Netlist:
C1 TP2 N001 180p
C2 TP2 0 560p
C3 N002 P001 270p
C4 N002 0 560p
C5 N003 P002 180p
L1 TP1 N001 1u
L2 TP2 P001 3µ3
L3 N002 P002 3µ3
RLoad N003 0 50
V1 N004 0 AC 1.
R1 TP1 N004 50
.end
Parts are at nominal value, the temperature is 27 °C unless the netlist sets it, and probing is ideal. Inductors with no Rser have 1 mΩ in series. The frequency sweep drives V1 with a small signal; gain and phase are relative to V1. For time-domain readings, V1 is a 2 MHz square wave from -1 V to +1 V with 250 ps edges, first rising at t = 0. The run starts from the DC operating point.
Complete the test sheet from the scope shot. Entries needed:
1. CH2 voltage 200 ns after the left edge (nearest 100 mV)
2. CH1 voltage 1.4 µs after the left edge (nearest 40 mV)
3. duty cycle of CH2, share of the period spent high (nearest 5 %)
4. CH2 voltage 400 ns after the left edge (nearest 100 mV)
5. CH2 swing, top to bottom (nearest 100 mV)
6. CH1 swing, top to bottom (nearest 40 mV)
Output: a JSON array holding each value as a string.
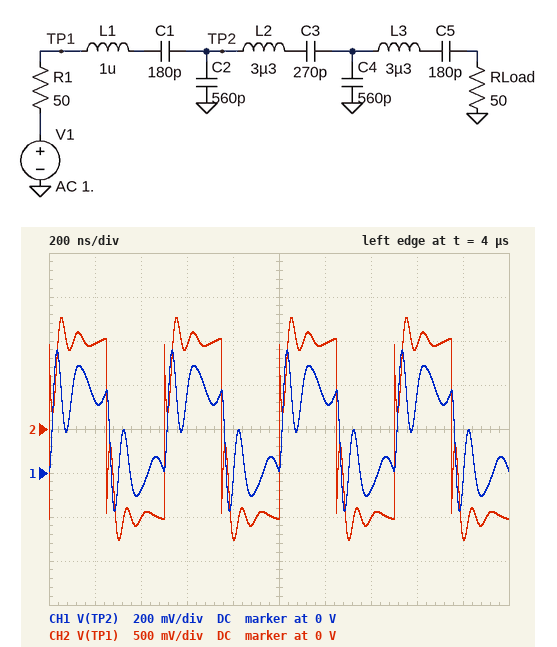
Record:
["1.0 V", "-80 mV", "50 %", "-1.0 V", "2.5 V", "720 mV"]
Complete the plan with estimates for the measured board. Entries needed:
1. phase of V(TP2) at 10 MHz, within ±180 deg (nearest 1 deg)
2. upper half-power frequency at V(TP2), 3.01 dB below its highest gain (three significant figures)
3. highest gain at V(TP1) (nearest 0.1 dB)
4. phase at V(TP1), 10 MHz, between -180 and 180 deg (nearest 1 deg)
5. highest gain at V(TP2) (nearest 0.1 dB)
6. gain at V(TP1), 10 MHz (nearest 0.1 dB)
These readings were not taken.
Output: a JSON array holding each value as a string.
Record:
["-38 deg", "15.6 MHz", "0 dB", "-38 deg", "-5.9 dB", "-2.1 dB"]
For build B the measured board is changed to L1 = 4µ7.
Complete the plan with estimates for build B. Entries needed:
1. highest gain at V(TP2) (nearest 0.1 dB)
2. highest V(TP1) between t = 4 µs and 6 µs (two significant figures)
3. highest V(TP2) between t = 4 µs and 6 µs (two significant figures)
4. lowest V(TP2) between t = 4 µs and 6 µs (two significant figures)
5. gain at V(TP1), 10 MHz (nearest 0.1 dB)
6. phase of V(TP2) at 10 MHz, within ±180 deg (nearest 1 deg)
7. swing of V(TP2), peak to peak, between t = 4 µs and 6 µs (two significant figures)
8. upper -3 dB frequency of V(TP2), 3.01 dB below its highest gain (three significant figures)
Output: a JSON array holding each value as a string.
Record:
["-3.0 dB", "1.3 V", "510 mV", "-130 mV", "-0.4 dB", "-163 deg", "640 mV", "8.77 MHz"]
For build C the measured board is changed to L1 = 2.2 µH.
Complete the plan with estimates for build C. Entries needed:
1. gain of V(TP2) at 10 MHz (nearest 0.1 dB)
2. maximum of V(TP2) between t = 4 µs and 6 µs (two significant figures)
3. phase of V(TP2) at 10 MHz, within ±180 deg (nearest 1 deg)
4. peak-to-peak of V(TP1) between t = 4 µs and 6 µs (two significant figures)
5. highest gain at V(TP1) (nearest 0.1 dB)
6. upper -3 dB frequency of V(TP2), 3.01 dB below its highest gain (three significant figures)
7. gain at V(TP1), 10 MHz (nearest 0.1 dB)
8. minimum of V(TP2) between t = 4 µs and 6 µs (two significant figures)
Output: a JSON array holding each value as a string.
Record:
["-2.7 dB", "600 mV", "-103 deg", "2.6 V", "0 dB", "10.4 MHz", "-12.8 dB", "-210 mV"]
